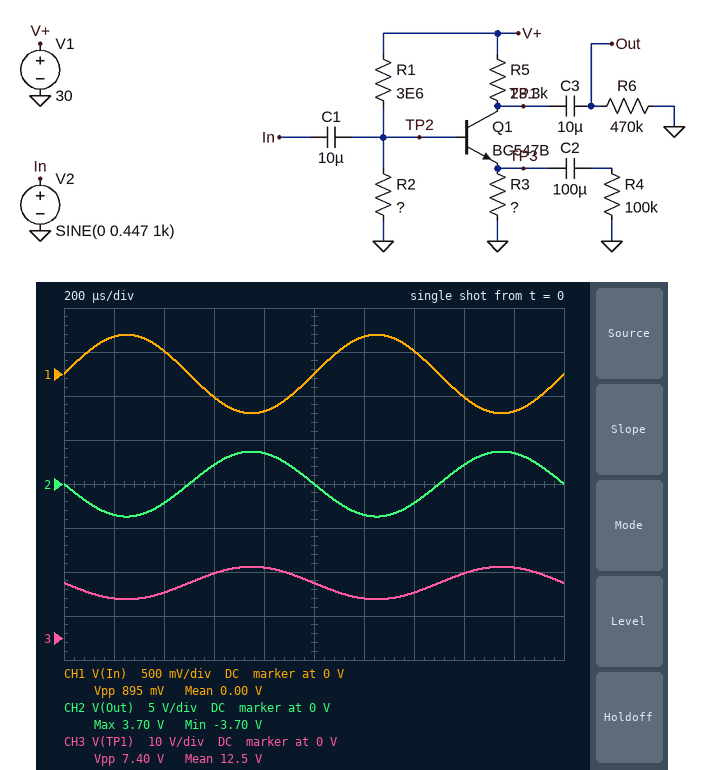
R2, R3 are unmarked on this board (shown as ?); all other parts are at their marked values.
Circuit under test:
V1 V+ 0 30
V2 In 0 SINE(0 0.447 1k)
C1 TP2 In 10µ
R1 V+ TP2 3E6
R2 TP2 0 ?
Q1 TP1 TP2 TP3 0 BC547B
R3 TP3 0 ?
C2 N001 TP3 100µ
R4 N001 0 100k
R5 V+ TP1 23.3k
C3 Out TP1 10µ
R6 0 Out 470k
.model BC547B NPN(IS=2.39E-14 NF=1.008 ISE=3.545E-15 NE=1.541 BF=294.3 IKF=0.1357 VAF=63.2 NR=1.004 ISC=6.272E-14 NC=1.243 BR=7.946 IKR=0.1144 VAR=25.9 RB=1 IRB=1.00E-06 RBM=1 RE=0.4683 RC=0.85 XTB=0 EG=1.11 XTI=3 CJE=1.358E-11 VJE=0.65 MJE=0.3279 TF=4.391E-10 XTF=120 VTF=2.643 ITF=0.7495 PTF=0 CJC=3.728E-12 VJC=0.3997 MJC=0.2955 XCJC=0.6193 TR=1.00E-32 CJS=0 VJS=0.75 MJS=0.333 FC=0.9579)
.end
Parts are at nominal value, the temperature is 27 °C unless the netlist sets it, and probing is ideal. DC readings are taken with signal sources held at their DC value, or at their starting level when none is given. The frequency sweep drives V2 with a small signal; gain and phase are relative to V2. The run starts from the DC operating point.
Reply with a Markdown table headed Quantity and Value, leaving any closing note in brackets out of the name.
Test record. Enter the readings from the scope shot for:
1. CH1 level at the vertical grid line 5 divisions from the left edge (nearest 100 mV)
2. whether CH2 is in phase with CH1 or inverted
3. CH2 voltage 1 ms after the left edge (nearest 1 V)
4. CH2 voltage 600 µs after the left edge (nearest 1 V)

| Quantity | Value |
|---|---|
| CH1 level at the vertical grid line 5 divisions from the left edge | 0 V |
| whether CH2 is in phase with CH1 or inverted | inverted |
| CH2 voltage 1 ms after the left edge | 0 V |
| CH2 voltage 600 µs after the left edge | 2 V |
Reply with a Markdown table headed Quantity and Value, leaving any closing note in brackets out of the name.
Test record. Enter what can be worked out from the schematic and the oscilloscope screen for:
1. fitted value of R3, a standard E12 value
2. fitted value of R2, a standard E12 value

| Quantity | Value |
|---|---|
| fitted value of R3, a standard E12 value | 2.7 kΩ |
| fitted value of R2, a standard E12 value | 390 kΩ |
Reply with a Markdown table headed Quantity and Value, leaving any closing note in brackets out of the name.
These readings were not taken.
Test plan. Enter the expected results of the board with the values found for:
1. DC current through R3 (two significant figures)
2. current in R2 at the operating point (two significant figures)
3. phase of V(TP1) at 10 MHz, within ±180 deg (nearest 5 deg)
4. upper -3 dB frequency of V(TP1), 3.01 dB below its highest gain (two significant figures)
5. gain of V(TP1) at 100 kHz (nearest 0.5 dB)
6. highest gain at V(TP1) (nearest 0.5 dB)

| Quantity | Value |
|---|---|
| DC current through R3 | 750 µA |
| current in R2 at the operating point | 6.8 µA |
| phase of V(TP1) at 10 MHz, within ±180 deg | 95 deg |
| upper -3 dB frequency of V(TP1), 3.01 dB below its highest gain | 5.1 MHz |
| gain of V(TP1) at 100 kHz | 18.5 dB |
| highest gain at V(TP1) | 18.5 dB |
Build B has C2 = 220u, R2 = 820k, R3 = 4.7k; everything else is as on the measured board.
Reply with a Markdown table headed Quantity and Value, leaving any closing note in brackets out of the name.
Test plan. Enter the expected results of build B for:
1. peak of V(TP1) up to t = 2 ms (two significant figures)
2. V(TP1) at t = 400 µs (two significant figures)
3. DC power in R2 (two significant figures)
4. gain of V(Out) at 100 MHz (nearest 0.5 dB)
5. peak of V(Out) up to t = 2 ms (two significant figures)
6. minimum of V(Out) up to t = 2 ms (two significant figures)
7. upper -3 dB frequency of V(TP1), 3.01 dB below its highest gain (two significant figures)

| Quantity | Value |
|---|---|
| peak of V(TP1) up to t = 2 ms | 12 V |
| V(TP1) at t = 400 µs | 8.8 V |
| DC power in R2 | 26 µW |
| gain of V(Out) at 100 MHz | 1.0 dB |
| peak of V(Out) up to t = 2 ms | 2.2 V |
| minimum of V(Out) up to t = 2 ms | -2.2 V |
| upper -3 dB frequency of V(TP1), 3.01 dB below its highest gain | 4.5 MHz |
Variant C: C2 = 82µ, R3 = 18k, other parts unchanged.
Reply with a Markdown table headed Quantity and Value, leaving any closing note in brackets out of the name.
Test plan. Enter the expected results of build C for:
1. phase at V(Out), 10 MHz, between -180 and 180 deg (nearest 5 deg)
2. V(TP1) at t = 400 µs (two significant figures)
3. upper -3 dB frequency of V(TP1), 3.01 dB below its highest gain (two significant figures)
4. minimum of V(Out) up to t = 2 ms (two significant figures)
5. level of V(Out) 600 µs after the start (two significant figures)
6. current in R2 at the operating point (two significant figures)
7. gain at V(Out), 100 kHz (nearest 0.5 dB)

| Quantity | Value |
|---|---|
| phase at V(Out), 10 MHz, between -180 and 180 deg | 65 deg |
| V(TP1) at t = 400 µs | 26 V |
| upper -3 dB frequency of V(TP1), 3.01 dB below its highest gain | 130 MHz |
| minimum of V(Out) up to t = 2 ms | -640 mV |
| level of V(Out) 600 µs after the start | 380 mV |
| current in R2 at the operating point | 8.5 µA |
| gain at V(Out), 100 kHz | 3.0 dB |
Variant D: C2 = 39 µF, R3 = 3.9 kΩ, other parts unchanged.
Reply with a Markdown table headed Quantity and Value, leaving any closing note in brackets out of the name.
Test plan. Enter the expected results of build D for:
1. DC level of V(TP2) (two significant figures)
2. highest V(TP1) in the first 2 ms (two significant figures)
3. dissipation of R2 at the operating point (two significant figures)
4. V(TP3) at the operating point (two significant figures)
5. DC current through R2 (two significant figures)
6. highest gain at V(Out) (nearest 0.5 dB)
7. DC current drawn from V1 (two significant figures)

| Quantity | Value |
|---|---|
| DC level of V(TP2) | 2.9 V |
| highest V(TP1) in the first 2 ms | 19 V |
| dissipation of R2 at the operating point | 21 µW |
| V(TP3) at the operating point | 2.3 V |
| DC current through R2 | 7.4 µA |
| highest gain at V(Out) | 15.5 dB |
| DC current drawn from V1 | 590 µA |
